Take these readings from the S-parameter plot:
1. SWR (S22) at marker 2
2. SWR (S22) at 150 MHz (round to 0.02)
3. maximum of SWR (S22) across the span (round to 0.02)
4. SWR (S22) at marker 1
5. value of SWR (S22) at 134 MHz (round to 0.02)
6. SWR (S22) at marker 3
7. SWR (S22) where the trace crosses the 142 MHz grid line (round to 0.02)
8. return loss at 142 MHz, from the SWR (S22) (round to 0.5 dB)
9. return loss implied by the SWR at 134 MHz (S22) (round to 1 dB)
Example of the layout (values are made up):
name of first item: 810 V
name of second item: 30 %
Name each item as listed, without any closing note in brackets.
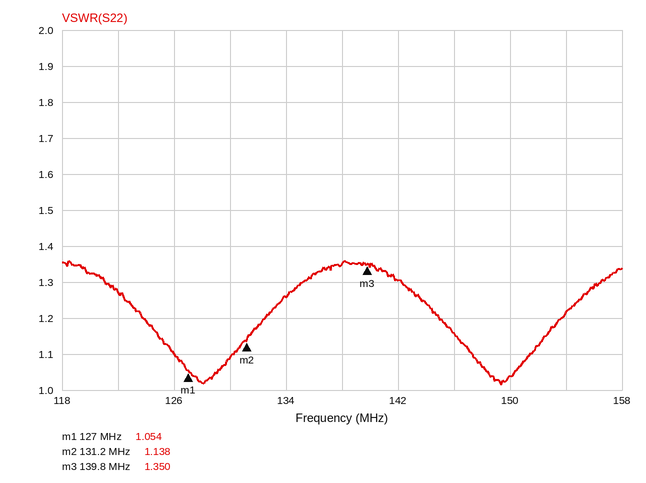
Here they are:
SWR (S22) at marker 2: 1.138
SWR (S22) at 150 MHz: 1.04
maximum of SWR (S22) across the span: 1.36
SWR (S22) at marker 1: 1.054
value of SWR (S22) at 134 MHz: 1.26
SWR (S22) at marker 3: 1.350
SWR (S22) where the trace crosses the 142 MHz grid line: 1.30
return loss at 142 MHz, from the SWR (S22): 17.5 dB
return loss implied by the SWR at 134 MHz (S22): 19 dB
